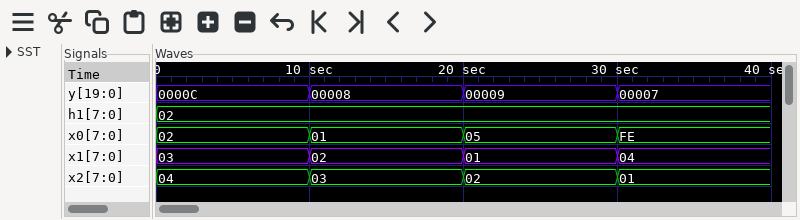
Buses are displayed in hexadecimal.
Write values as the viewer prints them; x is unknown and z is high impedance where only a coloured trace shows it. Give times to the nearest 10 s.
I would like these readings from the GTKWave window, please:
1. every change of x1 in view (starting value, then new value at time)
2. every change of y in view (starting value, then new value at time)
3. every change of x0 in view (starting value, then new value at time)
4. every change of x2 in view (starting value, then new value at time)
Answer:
03, 02 at 10 s, 01 at 20 s, 04 at 30 s
0000C, 00008 at 10 s, 00009 at 20 s, 00007 at 30 s
02, 01 at 10 s, 05 at 20 s, FE at 30 s
04, 03 at 10 s, 02 at 20 s, 01 at 30 s
